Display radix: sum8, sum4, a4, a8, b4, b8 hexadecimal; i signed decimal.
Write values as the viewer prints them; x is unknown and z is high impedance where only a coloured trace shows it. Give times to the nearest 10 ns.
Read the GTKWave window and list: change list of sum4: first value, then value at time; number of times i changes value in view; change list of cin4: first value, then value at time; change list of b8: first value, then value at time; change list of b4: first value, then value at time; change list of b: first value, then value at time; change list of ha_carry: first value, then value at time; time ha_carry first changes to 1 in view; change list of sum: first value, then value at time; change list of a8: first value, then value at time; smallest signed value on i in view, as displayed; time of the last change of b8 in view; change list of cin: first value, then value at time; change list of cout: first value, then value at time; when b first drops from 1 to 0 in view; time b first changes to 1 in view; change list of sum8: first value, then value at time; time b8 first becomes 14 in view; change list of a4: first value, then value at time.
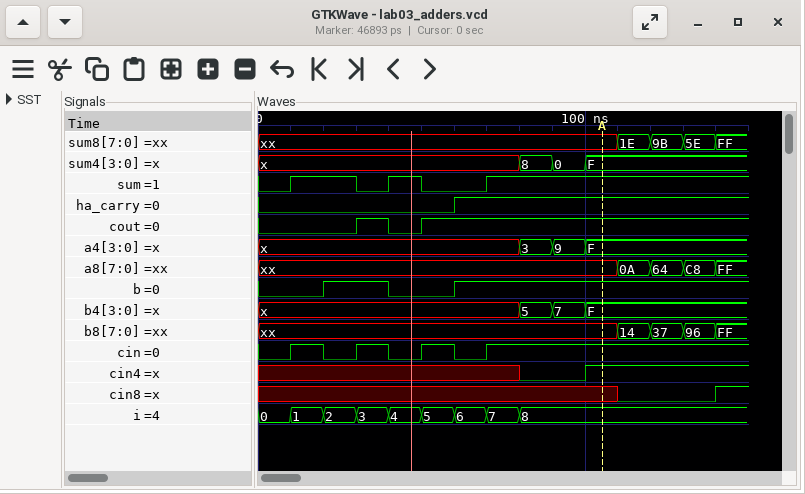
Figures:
x, 8 at 80 ns, 0 at 90 ns, F at 100 ns
8
x, 0 at 80 ns, 1 at 100 ns
xx, 14 at 110 ns, 37 at 120 ns, 96 at 130 ns, FF at 140 ns
x, 5 at 80 ns, 7 at 90 ns, F at 100 ns
0, 1 at 20 ns, 0 at 40 ns, 1 at 60 ns
0, 1 at 60 ns
60 ns
0, 1 at 10 ns, 0 at 30 ns, 1 at 40 ns, 0 at 50 ns, 1 at 70 ns
xx, 0A at 110 ns, 64 at 120 ns, C8 at 130 ns, FF at 140 ns
0
140 ns
0, 1 at 10 ns, 0 at 20 ns, 1 at 30 ns, 0 at 40 ns, 1 at 50 ns, 0 at 60 ns, 1 at 70 ns
0, 1 at 30 ns, 0 at 40 ns, 1 at 50 ns
40 ns
20 ns
xx, 1E at 110 ns, 9B at 120 ns, 5E at 130 ns, FF at 140 ns
110 ns
x, 3 at 80 ns, 9 at 90 ns, F at 100 ns
